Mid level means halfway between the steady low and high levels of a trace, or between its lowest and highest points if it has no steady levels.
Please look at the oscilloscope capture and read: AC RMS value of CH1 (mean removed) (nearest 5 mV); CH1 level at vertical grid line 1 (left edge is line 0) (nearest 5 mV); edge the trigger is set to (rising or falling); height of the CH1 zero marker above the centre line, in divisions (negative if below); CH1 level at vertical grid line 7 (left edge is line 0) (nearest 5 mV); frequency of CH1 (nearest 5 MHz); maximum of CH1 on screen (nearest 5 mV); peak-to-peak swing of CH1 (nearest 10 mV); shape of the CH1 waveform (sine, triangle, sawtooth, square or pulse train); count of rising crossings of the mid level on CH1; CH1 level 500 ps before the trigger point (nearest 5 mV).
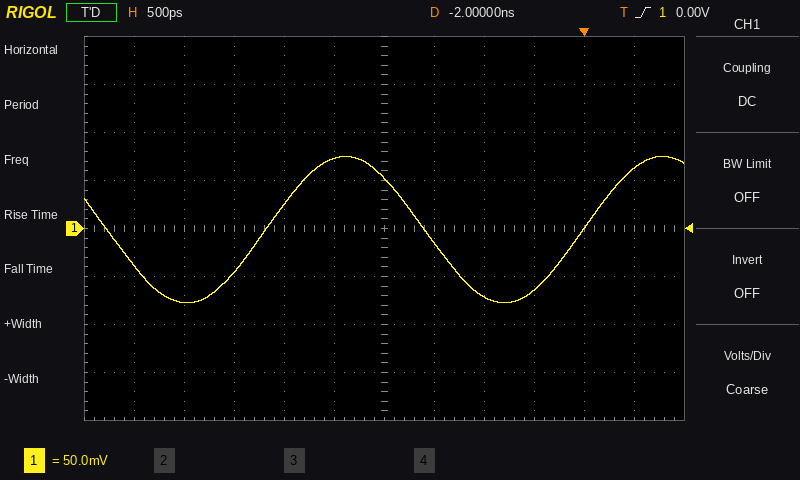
55 mV
-40 mV
rising
0.0 div
-15 mV
315 MHz
75 mV
150 mV
sine
2
-65 mV
